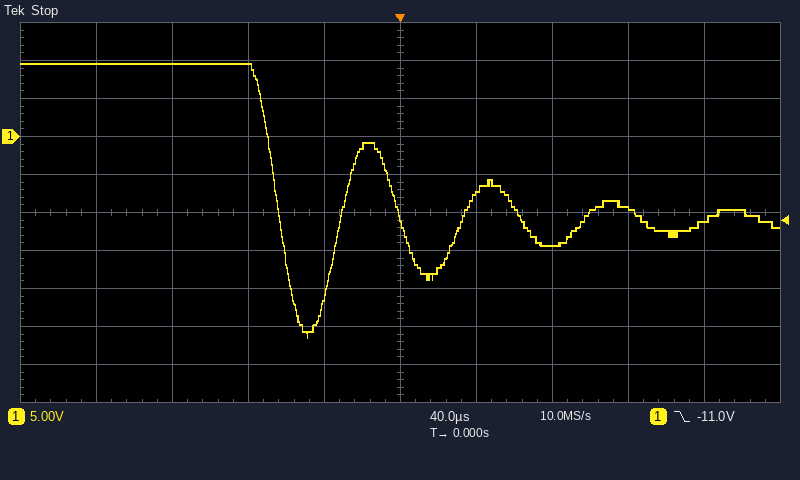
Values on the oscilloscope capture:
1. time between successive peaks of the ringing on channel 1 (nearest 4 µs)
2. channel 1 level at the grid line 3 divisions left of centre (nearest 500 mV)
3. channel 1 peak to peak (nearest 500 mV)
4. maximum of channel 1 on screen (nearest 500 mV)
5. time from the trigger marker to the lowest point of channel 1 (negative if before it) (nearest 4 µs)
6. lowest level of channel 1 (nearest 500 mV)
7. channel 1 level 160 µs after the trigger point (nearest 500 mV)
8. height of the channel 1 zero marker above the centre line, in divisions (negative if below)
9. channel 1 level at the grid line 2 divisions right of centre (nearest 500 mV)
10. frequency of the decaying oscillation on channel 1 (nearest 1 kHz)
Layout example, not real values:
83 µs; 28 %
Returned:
64 µs; 9.5 V; 36.0 V; 9.5 V; -48 µs; -26.5 V; -11.0 V; +2.0 div; -14.5 V; 16 kHz
